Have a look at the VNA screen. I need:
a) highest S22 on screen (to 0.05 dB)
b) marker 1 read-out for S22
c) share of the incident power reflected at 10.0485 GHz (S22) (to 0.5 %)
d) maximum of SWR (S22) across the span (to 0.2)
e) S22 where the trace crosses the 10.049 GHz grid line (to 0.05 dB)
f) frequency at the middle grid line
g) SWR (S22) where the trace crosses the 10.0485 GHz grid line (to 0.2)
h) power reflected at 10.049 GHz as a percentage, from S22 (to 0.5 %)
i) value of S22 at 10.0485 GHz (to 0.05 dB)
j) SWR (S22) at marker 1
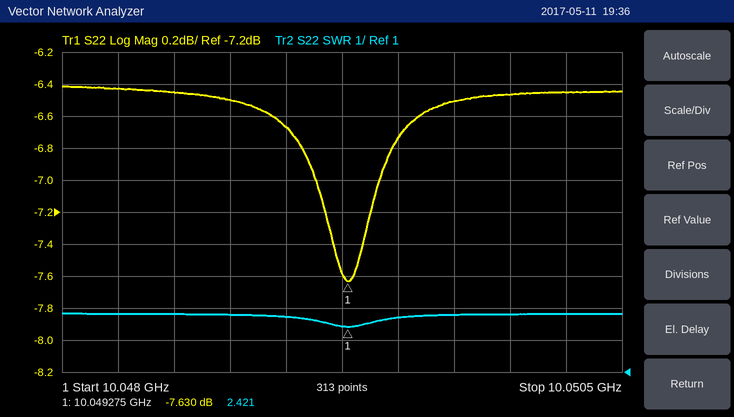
-6.40 dB
-7.630 dB
22.5 %
2.8
-6.65 dB
10.04925 GHz
2.8
21.5 %
-6.45 dB
2.421
